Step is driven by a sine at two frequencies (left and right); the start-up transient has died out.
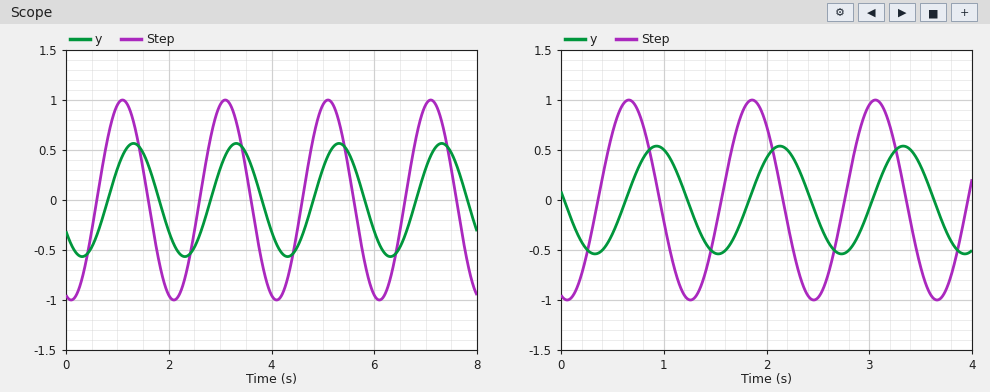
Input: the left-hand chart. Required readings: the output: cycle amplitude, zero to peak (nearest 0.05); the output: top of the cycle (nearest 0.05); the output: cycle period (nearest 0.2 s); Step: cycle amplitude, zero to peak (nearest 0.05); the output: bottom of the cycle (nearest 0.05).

0.55
0.55
2.0 s
1.00
-0.55
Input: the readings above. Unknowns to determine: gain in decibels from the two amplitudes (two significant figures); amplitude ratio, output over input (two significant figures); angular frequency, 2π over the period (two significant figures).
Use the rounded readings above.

-5.2 dB
0.55
3.1 rad/s
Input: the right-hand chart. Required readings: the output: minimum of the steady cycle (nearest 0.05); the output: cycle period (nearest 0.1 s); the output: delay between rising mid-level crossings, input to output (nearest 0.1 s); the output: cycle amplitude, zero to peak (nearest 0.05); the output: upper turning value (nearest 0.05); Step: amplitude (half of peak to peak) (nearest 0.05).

-0.55
1.2 s
0.3 s
0.55
0.55
1.00
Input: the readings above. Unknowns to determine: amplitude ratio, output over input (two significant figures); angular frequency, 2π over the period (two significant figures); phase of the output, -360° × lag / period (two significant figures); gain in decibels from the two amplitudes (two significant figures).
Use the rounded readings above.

0.55
5.2 rad/s
-90°
-5.2 dB
